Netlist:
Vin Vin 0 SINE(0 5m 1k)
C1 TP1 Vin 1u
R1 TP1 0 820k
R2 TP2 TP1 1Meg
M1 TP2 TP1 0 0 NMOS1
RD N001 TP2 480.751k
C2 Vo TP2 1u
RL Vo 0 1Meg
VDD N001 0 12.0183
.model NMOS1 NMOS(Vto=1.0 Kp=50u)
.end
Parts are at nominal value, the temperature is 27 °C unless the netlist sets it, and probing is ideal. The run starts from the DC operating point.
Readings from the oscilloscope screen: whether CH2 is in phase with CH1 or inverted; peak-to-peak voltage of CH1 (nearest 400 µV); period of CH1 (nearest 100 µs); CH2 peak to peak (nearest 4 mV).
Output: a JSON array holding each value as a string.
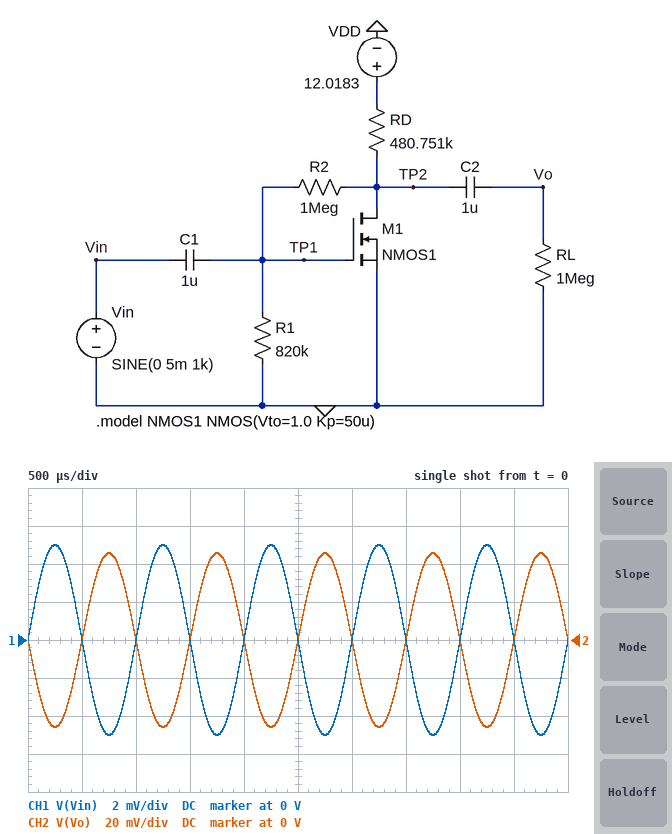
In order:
["inverted", "10.0 mV", "1.0 ms", "92 mV"]
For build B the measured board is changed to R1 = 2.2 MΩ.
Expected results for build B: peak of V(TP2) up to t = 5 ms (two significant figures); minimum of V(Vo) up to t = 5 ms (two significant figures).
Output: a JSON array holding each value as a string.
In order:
["2.8 V", "-52 mV"]
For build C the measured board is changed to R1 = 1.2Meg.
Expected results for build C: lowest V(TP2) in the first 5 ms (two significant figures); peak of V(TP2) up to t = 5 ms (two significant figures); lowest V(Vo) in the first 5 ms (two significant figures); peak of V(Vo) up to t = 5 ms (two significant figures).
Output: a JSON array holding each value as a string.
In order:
["3.3 V", "3.4 V", "-49 mV", "49 mV"]
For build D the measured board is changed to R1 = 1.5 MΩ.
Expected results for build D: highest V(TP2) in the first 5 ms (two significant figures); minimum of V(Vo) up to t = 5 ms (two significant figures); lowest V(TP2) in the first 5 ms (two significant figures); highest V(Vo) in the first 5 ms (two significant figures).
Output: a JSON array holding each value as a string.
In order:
["3.1 V", "-50 mV", "3.0 V", "50 mV"]
